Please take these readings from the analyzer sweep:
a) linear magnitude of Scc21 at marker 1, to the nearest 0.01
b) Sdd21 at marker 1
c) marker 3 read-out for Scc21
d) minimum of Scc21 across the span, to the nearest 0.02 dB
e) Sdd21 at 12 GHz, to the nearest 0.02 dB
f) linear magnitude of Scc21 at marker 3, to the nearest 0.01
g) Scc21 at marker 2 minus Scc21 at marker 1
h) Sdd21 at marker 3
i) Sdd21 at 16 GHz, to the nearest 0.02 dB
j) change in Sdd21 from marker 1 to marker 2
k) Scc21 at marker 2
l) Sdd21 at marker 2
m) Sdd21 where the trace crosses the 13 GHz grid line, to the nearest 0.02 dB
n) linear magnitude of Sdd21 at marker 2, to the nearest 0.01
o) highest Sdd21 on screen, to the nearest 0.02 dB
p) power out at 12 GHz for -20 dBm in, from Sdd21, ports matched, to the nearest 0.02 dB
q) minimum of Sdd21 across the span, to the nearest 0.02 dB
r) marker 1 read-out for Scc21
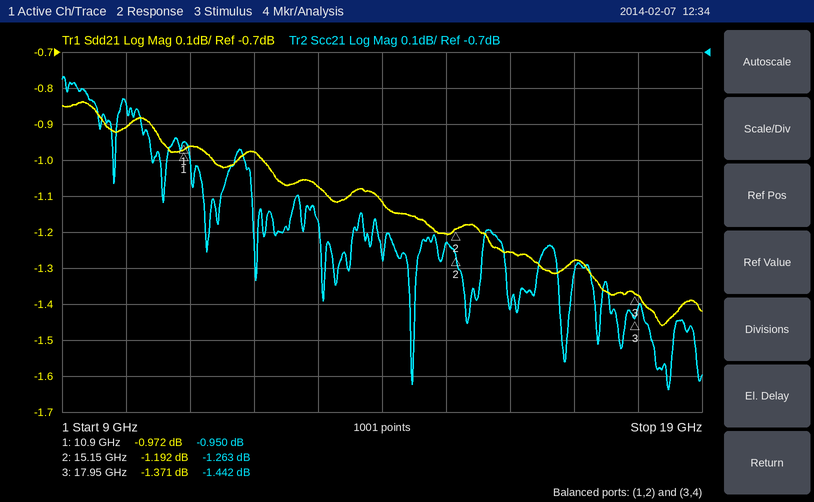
0.90
-0.972 dB
-1.442 dB
-1.64 dB
-0.98 dB
0.85
-0.313 dB
-1.371 dB
-1.26 dB
-0.220 dB
-1.263 dB
-1.192 dB
-1.08 dB
0.87
-0.84 dB
-20.98 dBm
-1.46 dB
-0.950 dB
